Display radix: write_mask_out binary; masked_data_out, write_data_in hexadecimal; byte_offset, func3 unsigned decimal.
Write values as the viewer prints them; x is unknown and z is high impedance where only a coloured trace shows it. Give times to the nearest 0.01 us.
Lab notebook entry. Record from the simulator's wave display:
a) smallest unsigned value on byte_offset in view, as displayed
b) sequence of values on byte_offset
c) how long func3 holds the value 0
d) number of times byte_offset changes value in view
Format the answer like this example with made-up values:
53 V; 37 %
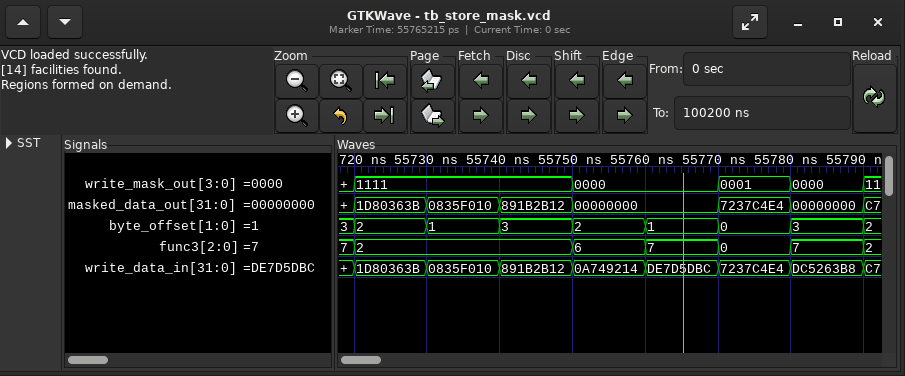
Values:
0; 3, 2, 1, 3, 2, 1, 0, 3, 2; 0.01 us; 8
